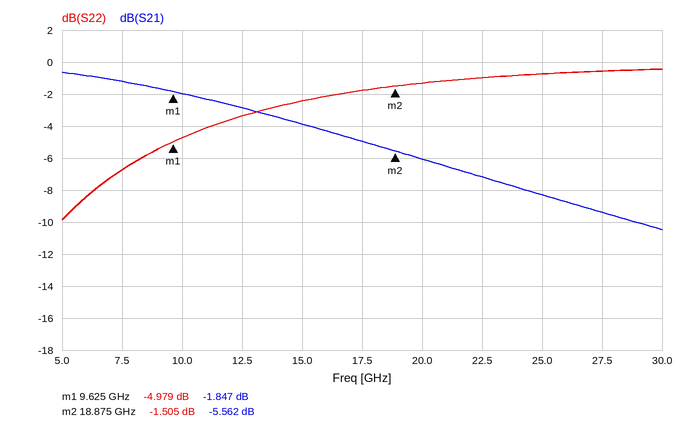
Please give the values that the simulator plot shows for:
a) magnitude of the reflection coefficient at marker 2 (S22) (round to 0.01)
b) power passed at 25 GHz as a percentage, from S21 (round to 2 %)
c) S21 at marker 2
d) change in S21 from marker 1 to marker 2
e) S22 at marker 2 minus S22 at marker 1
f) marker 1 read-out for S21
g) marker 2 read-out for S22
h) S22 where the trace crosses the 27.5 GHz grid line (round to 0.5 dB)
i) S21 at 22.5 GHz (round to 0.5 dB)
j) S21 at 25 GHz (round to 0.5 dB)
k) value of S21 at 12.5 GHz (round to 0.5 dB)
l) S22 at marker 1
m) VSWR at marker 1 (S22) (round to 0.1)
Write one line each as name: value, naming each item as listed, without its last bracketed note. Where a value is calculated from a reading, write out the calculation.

magnitude of the reflection coefficient at marker 2 (S22): 10^(-1.505/20) ≈ 0.84
power passed at 25 GHz as a percentage, from S21: 10^(-8.5/10) ≈ 14 %
S21 at marker 2: -5.562 dB
change in S21 from marker 1 to marker 2: -5.562 − (-1.847) = -3.715 dB
S22 at marker 2 minus S22 at marker 1: -1.505 − (-4.979) = 3.474 dB
marker 1 read-out for S21: -1.847 dB
marker 2 read-out for S22: -1.505 dB
S22 where the trace crosses the 27.5 GHz grid line: -0.5 dB
S21 at 22.5 GHz: -7.0 dB
S21 at 25 GHz: -8.5 dB
value of S21 at 12.5 GHz: -3.0 dB
S22 at marker 1: -4.979 dB
VSWR at marker 1 (S22): (1 + 0.5637)/(1 − 0.5637) ≈ 3.6
